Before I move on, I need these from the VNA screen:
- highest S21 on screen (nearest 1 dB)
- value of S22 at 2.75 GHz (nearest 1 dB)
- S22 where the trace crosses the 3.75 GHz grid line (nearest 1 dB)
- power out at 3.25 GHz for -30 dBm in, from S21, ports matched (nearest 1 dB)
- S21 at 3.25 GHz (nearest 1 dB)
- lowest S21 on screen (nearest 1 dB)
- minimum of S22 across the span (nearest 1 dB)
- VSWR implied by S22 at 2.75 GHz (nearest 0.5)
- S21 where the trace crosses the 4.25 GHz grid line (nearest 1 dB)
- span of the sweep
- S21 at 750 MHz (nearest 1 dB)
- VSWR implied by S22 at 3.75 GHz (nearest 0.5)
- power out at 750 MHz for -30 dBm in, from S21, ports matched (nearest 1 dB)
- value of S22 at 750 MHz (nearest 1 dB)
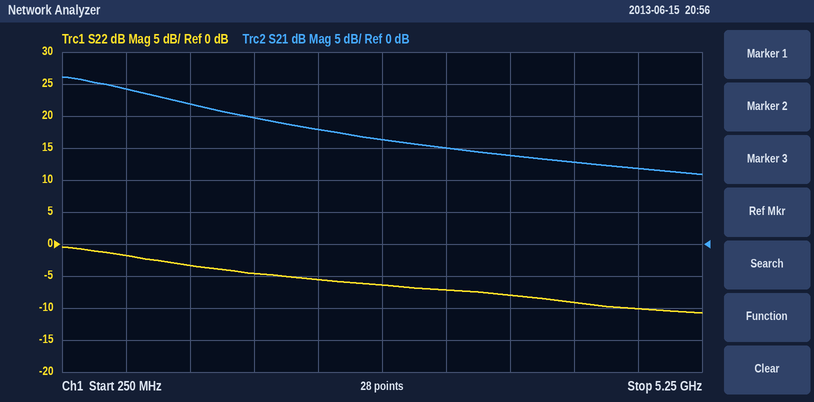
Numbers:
26 dB
-6 dB
-8 dB
-15 dBm
15 dB
11 dB
-11 dB
3.0
13 dB
5 GHz
24 dB
2.5
-6 dBm
-2 dB
